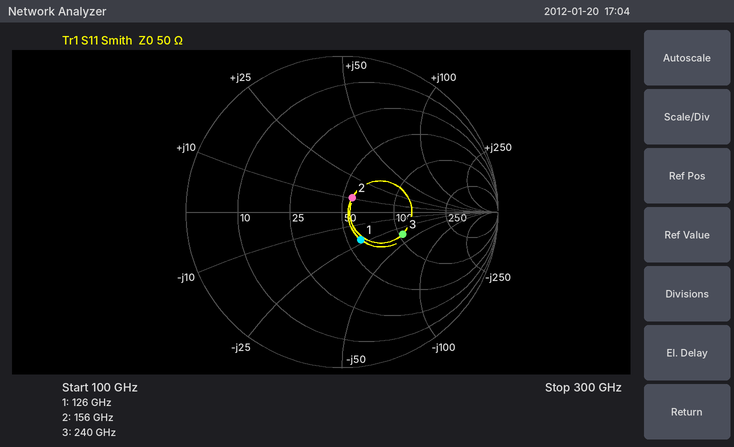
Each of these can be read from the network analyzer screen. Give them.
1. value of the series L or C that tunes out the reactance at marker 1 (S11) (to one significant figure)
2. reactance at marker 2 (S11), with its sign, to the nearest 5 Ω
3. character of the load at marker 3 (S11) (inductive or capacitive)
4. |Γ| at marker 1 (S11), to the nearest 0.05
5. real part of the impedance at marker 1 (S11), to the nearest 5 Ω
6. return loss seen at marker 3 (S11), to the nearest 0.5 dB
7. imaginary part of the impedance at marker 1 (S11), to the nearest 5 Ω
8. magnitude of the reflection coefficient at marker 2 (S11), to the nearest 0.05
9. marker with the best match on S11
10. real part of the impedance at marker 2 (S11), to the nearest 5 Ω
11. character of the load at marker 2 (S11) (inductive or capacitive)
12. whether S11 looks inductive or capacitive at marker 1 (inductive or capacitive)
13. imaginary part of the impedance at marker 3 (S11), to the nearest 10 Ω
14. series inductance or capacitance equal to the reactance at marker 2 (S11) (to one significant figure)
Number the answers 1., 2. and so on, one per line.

1. 30 pH
2. +10 Ω
3. capacitive
4. 0.20
5. 60 Ω
6. 7.5 dB
7. -20 Ω
8. 0.10
9. marker 2
10. 55 Ω
11. inductive
12. capacitive
13. -40 Ω
14. 10 pH
